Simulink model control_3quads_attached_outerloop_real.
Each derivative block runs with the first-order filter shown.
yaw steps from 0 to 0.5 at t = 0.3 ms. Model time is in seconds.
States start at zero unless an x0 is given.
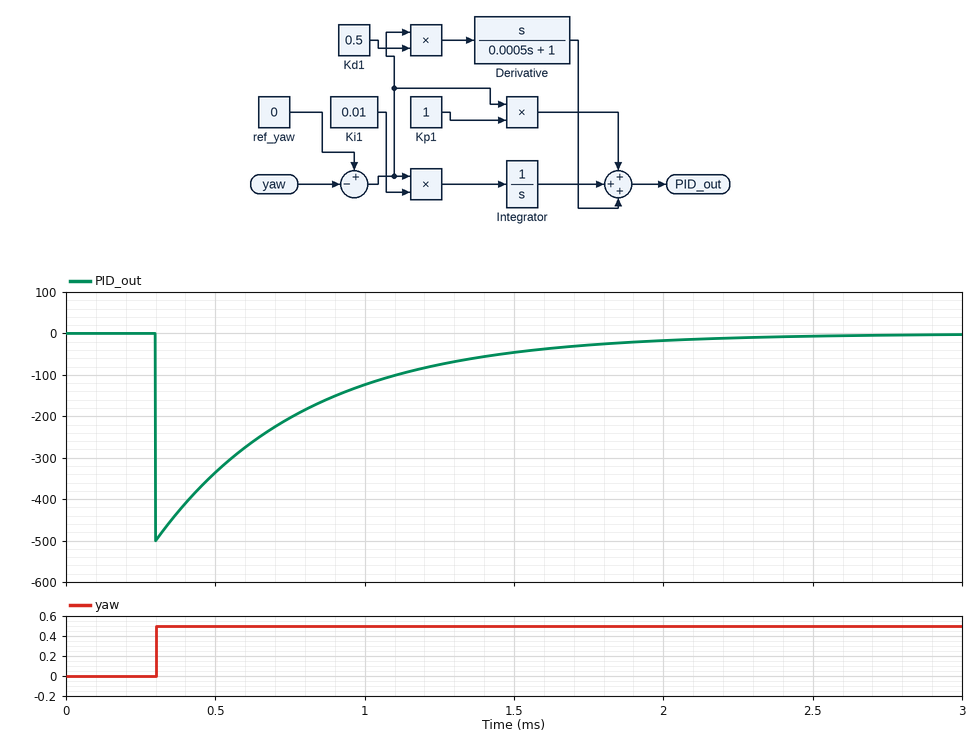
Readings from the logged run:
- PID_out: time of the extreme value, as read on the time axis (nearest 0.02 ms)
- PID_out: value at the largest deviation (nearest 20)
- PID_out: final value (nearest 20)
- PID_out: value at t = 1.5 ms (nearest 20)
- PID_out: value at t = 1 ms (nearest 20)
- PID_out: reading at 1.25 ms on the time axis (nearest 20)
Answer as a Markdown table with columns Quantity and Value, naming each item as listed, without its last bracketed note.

| Quantity | Value |
|---|---|
| PID_out: time of the extreme value, as read on the time axis | 0.30 ms |
| PID_out: value at the largest deviation | -500 |
| PID_out: final value | 0 |
| PID_out: value at t = 1.5 ms | -40 |
| PID_out: value at t = 1 ms | -120 |
| PID_out: reading at 1.25 ms on the time axis | -80 |
